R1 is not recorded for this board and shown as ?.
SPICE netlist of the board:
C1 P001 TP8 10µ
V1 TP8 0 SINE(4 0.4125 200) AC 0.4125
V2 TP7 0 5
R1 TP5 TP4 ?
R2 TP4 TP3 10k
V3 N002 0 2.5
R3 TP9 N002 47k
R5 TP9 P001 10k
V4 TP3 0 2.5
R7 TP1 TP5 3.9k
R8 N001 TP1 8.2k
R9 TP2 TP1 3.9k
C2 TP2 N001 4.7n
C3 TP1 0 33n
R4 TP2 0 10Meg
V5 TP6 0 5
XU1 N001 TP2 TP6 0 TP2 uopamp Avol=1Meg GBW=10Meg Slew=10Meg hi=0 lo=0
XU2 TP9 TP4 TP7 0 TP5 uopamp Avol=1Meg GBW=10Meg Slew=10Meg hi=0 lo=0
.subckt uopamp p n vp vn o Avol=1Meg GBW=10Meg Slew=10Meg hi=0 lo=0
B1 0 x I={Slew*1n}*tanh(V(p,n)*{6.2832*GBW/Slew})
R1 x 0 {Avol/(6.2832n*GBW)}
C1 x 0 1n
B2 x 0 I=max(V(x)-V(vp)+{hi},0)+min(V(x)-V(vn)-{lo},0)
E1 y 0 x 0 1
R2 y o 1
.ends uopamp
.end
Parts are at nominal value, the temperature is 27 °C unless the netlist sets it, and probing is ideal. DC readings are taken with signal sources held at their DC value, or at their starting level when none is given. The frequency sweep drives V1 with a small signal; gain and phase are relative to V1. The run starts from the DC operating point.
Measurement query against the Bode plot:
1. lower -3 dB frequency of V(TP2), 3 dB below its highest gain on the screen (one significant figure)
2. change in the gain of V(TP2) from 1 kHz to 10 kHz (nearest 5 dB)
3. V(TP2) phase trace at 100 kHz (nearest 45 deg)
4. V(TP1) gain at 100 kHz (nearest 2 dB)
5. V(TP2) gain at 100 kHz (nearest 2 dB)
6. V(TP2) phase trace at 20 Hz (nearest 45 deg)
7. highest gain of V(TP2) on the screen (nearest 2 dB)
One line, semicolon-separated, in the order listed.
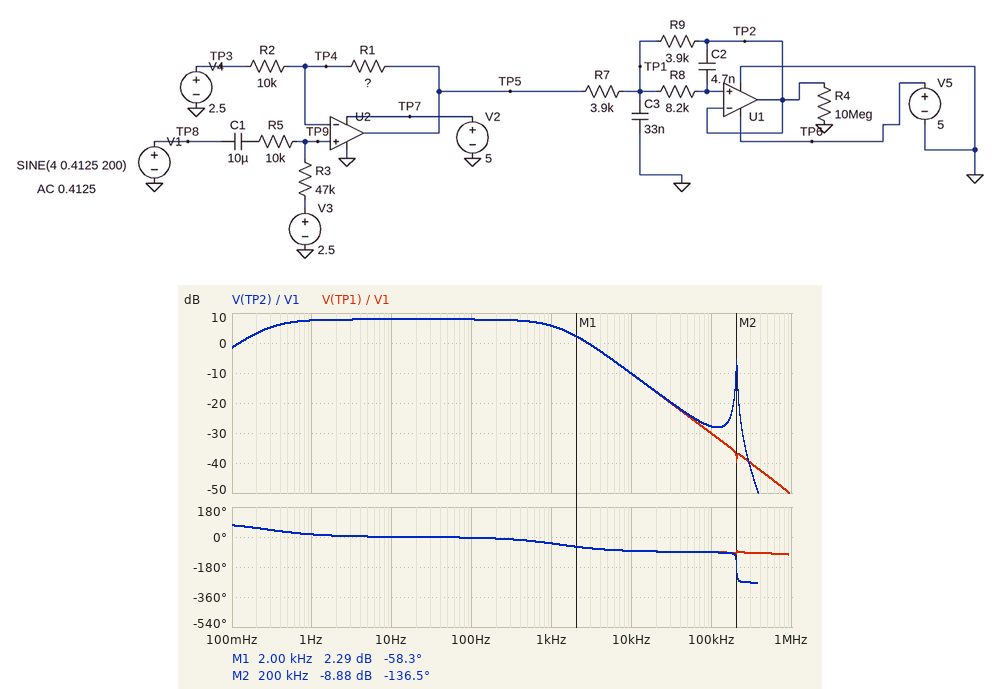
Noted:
300 mHz; -15 dB; -90 deg; -30 dB; -28 dB; 0 deg; 8 dB
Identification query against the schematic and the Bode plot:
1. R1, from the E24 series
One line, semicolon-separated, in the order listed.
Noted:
20 kΩ
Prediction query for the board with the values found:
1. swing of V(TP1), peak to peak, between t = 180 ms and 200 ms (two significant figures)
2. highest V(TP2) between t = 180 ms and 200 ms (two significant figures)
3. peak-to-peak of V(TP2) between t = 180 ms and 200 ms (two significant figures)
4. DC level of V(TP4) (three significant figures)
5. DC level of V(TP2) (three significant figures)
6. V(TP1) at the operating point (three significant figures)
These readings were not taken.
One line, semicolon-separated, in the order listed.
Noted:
2.0 V; 3.5 V; 2.0 V; 2.50 V; 2.50 V; 2.50 V
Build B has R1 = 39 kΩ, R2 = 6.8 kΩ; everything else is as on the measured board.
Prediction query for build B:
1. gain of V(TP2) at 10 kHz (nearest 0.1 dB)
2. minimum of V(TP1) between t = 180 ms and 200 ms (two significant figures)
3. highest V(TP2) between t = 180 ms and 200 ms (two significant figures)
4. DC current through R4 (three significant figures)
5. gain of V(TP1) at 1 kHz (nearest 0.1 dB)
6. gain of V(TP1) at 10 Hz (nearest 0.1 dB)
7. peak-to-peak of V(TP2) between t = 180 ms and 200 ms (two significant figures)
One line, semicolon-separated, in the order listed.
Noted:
-3.3 dB; 240 mV; 4.8 V; 250 nA; 12.7 dB; 14.9 dB; 4.5 V
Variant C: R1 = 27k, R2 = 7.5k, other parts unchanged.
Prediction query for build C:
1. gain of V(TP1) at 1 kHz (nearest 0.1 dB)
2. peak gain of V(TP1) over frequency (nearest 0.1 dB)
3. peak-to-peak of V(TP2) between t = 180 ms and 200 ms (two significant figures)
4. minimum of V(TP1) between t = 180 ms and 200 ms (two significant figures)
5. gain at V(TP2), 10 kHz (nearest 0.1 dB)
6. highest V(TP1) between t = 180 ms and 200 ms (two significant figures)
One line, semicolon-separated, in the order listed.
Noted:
9.4 dB; 11.6 dB; 3.1 V; 950 mV; -6.6 dB; 4.0 V
